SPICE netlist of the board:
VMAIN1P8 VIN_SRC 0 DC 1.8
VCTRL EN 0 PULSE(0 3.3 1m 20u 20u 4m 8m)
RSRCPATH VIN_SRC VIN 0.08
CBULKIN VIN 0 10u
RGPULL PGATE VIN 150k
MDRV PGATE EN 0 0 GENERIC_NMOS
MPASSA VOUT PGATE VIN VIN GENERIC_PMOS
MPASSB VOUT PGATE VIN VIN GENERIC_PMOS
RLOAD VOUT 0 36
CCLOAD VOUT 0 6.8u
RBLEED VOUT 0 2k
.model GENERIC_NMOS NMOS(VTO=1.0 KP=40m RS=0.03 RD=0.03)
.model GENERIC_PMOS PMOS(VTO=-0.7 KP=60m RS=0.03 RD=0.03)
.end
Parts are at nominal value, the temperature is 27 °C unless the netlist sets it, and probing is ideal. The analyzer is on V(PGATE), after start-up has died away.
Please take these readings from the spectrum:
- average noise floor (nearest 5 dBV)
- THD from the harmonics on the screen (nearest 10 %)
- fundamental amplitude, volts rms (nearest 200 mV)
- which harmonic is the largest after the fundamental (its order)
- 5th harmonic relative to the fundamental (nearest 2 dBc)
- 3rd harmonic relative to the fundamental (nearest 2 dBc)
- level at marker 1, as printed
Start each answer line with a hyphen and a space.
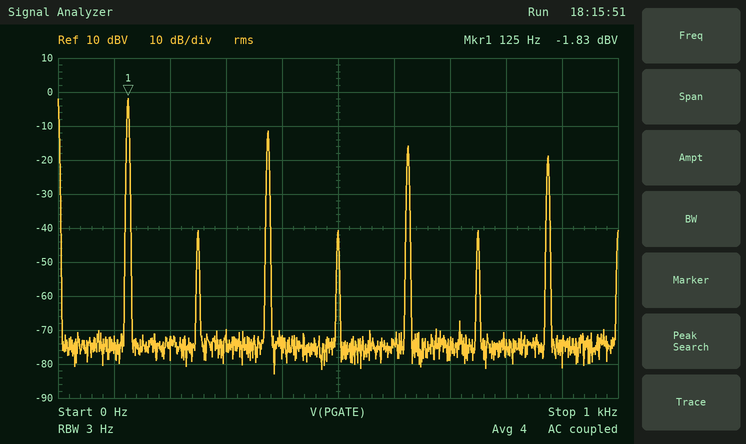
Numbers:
- -75 dBV
- 40 %
- 800 mV
- 3
- -14 dBc
- -10 dBc
- -1.83 dBV
